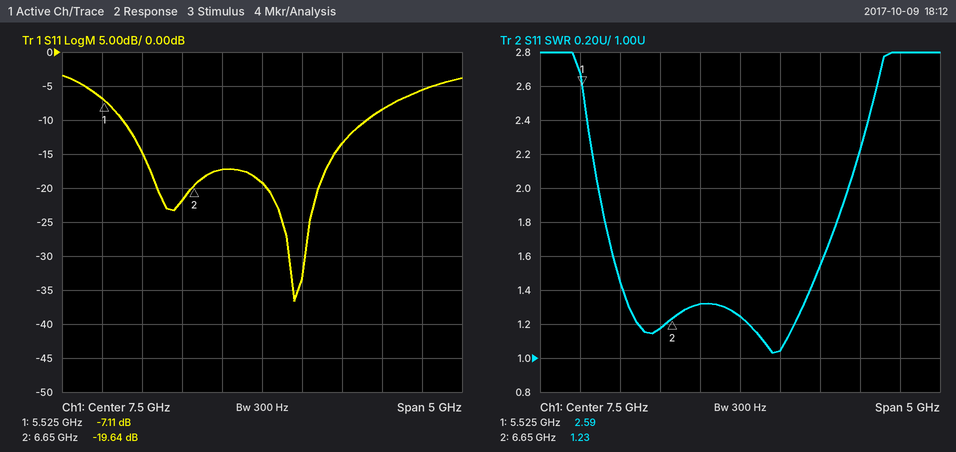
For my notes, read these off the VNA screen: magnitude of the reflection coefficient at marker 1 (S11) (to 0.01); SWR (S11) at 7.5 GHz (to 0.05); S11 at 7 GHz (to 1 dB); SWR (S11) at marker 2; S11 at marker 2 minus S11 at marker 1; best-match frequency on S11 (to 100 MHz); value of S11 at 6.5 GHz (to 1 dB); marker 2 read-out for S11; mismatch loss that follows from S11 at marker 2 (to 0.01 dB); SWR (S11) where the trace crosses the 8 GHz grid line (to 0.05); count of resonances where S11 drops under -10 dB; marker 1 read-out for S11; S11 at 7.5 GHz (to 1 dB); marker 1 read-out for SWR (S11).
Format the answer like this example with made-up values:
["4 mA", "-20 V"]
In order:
["0.44", "1.25", "-17 dB", "1.23", "-12.53 dB", "7.9 GHz", "-22 dB", "-19.64 dB", "0.05 dB", "1.05", "2", "-7.11 dB", "-19 dB", "2.59"]
